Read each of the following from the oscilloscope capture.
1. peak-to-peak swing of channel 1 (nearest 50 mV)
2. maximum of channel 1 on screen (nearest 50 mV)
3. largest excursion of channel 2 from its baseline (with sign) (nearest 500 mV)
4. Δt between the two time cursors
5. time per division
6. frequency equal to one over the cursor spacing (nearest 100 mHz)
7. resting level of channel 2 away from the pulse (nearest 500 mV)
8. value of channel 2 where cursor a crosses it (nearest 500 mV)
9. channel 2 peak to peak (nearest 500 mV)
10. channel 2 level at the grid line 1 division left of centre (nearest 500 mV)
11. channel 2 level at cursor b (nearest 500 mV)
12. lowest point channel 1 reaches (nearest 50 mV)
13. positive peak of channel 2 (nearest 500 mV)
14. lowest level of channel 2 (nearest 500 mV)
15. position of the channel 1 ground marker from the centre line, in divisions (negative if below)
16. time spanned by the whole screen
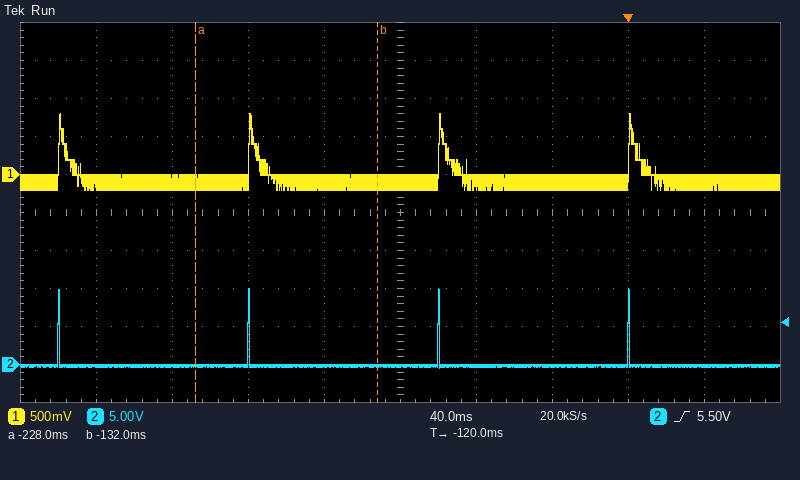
1.00 V
800 mV
+10.0 V
96 ms
40 ms
10.4 Hz
0.0 V
0.0 V
10.5 V
0.0 V
0.0 V
-200 mV
10.0 V
-500 mV
+1.0 div
400 ms
